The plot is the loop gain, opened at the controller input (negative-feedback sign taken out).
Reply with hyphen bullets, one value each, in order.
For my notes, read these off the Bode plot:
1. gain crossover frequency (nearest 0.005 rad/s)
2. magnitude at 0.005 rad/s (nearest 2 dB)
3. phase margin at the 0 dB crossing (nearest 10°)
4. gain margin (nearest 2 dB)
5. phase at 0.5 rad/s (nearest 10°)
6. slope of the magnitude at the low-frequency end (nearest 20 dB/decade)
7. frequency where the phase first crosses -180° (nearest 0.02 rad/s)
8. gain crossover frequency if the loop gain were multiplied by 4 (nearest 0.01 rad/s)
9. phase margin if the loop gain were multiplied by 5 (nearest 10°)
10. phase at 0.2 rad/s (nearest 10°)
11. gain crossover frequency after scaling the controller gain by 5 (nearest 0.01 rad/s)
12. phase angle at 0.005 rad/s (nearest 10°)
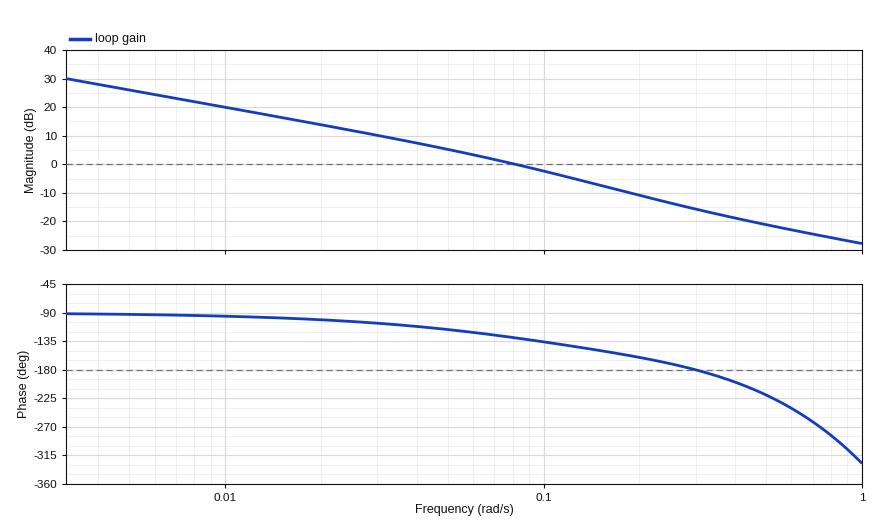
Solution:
- 0.080 rad/s
- 26 dB
- 50°
- 16 dB
- -220°
- -20 dB/decade
- 0.30 rad/s
- 0.22 rad/s
- 10°
- -160°
- 0.26 rad/s
- -90°
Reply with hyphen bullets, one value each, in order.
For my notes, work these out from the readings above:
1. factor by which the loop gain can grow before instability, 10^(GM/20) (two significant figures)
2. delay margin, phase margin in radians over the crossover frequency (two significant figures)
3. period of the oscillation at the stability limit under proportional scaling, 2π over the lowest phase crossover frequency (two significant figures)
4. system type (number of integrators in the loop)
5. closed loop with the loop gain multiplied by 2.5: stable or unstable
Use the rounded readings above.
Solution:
- 6.3
- 11 s
- 21 s
- 1
- stable
